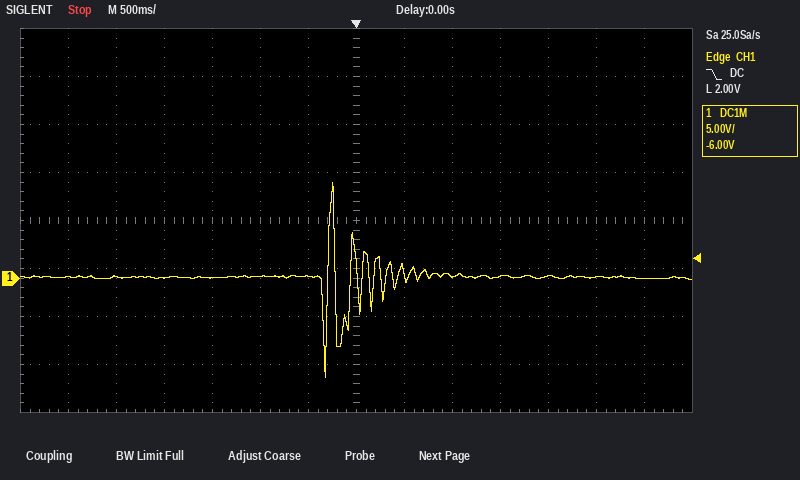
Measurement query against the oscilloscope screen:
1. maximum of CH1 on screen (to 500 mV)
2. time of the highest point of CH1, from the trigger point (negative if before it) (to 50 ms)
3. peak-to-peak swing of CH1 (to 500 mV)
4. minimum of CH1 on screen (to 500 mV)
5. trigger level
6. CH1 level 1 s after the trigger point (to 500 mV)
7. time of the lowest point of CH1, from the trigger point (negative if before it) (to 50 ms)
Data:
10.0 V
-250 ms
20.5 V
-10.5 V
2.00 V
0.0 V
-300 ms
